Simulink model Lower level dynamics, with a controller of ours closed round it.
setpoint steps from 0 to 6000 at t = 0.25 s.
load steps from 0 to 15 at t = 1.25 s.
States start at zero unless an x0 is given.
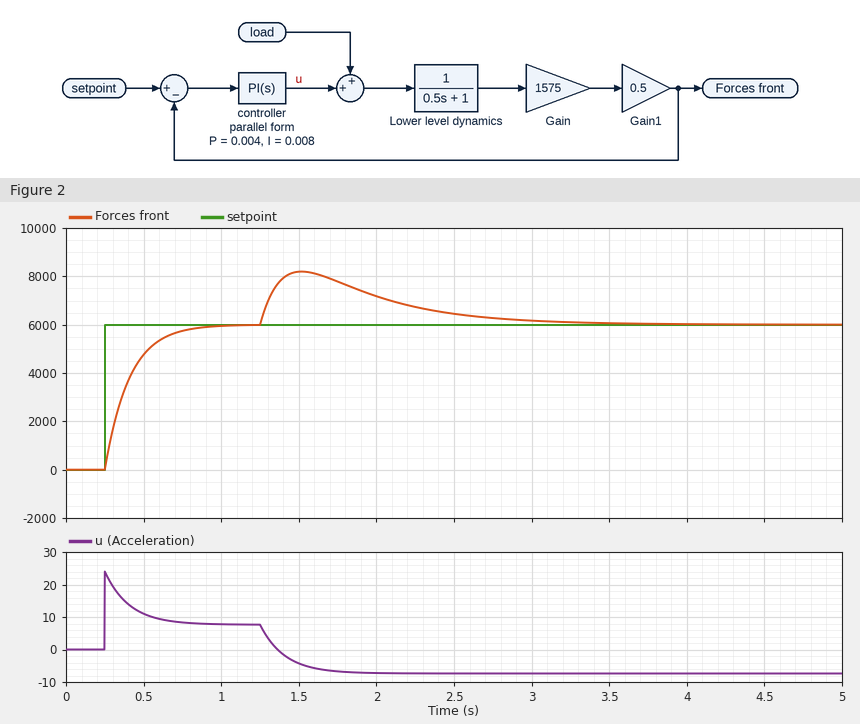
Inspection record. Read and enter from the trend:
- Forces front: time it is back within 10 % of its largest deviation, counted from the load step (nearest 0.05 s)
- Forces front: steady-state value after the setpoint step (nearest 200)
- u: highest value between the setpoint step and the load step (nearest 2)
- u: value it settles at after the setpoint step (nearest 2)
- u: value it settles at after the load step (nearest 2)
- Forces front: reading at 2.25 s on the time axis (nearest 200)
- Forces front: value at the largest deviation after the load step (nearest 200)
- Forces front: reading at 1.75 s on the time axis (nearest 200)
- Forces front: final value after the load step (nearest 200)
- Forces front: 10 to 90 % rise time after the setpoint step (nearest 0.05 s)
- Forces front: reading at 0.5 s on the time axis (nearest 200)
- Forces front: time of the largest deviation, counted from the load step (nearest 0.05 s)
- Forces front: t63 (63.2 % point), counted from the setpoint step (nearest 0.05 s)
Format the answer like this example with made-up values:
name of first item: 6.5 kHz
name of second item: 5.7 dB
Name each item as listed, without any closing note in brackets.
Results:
Forces front: time it is back within 10 % of its largest deviation, counted from the load step: 1.60 s
Forces front: steady-state value after the setpoint step: 6000
u: highest value between the setpoint step and the load step: 24
u: value it settles at after the setpoint step: 8
u: value it settles at after the load step: -8
Forces front: reading at 2.25 s on the time axis: 6800
Forces front: value at the largest deviation after the load step: 8200
Forces front: reading at 1.75 s on the time axis: 7800
Forces front: final value after the load step: 6000
Forces front: 10 to 90 % rise time after the setpoint step: 0.35 s
Forces front: reading at 0.5 s on the time axis: 4800
Forces front: time of the largest deviation, counted from the load step: 0.25 s
Forces front: t63 (63.2 % point), counted from the setpoint step: 0.15 s
